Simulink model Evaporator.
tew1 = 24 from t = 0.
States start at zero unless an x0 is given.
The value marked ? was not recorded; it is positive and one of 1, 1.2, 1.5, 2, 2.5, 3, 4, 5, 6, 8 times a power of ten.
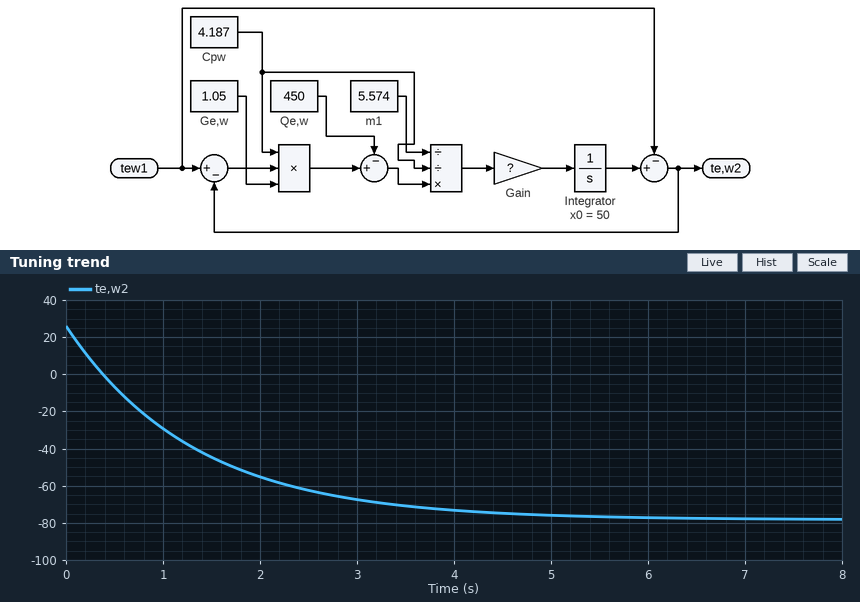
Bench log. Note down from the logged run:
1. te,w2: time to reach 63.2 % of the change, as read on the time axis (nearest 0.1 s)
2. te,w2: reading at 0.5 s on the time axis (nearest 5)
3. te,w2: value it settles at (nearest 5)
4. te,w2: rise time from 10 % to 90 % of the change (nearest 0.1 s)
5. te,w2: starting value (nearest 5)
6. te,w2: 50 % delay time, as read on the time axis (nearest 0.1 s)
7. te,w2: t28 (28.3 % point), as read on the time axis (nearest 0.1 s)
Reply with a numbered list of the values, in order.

1. 1.3 s
2. -5
3. -80
4. 2.9 s
5. 25
6. 0.9 s
7. 0.4 s
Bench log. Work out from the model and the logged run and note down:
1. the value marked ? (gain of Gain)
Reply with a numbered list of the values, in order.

1. 4
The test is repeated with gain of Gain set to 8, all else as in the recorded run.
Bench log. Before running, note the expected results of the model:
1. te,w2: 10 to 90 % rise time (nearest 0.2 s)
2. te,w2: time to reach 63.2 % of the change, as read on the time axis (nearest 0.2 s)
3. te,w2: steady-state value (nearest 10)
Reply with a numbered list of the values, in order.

1. 1.4 s
2. 0.6 s
3. -80
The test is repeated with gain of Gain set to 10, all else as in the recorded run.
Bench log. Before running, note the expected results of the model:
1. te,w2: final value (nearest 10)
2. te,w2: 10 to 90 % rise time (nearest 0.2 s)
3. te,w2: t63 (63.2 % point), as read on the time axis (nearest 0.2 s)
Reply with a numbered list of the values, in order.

1. -80
2. 1.2 s
3. 0.6 s
